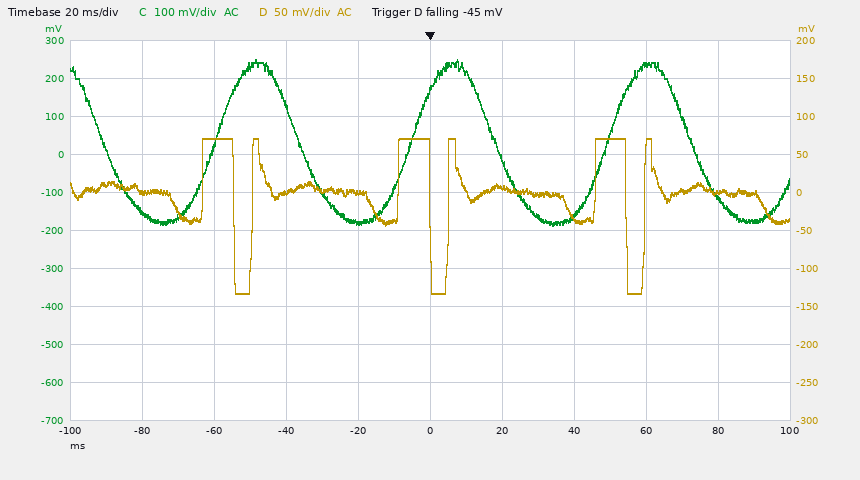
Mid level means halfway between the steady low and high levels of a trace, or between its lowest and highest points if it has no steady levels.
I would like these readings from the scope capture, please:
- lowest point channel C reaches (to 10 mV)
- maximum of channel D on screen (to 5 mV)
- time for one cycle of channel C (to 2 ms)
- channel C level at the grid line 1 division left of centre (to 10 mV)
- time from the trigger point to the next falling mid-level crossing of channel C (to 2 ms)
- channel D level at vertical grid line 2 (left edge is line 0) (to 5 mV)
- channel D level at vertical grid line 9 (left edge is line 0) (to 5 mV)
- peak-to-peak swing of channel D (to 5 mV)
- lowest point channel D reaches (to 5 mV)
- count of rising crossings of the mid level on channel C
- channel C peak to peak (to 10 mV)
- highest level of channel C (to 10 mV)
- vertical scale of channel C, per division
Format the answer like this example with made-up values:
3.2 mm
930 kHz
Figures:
-190 mV
70 mV
54 ms
-180 mV
18 ms
70 mV
0 mV
205 mV
-135 mV
3
440 mV
250 mV
100 mV
